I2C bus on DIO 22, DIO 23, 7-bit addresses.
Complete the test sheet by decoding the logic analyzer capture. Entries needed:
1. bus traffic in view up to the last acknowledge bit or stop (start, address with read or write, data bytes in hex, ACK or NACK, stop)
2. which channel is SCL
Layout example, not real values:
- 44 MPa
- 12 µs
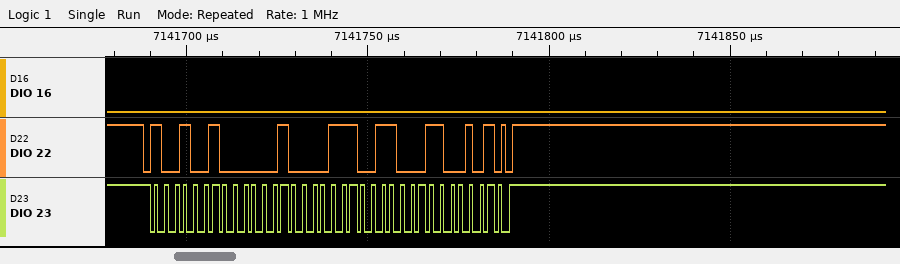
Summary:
- start, address 49 write ACK, 08 ACK, E6 ACK, 65 ACK, stop
- DIO 23
